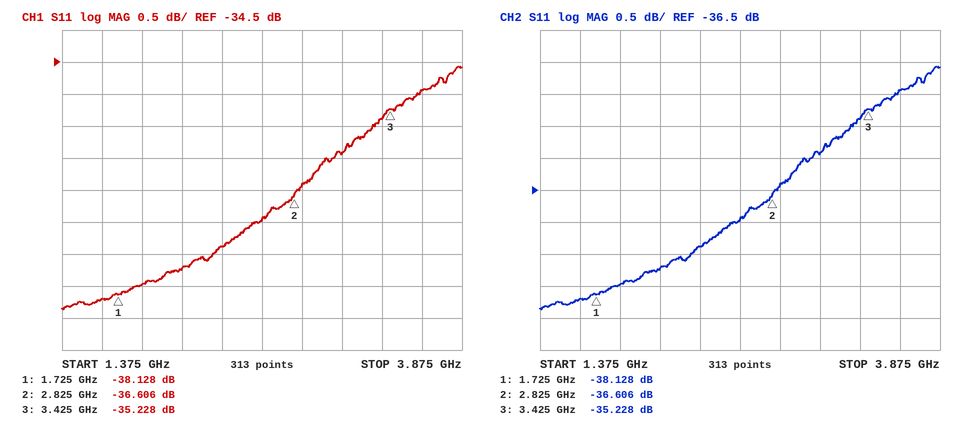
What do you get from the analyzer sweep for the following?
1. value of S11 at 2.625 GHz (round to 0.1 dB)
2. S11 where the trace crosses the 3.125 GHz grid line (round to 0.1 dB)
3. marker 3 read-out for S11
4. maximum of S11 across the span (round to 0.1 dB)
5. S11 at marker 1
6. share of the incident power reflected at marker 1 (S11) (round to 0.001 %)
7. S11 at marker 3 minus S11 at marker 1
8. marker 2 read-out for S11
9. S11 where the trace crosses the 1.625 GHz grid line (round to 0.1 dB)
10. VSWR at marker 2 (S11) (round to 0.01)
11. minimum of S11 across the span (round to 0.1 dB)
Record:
-37.0 dB
-35.9 dB
-35.228 dB
-34.6 dB
-38.128 dB
0.015 %
2.900 dB
-36.606 dB
-38.2 dB
1.03
-38.4 dB
